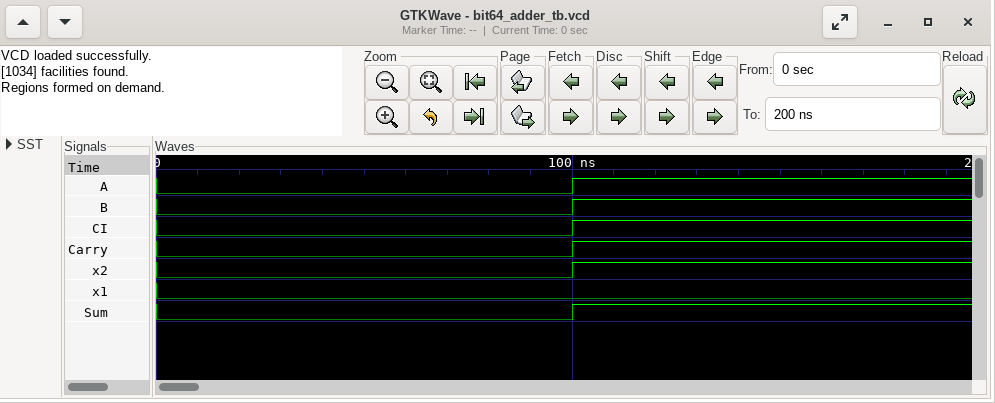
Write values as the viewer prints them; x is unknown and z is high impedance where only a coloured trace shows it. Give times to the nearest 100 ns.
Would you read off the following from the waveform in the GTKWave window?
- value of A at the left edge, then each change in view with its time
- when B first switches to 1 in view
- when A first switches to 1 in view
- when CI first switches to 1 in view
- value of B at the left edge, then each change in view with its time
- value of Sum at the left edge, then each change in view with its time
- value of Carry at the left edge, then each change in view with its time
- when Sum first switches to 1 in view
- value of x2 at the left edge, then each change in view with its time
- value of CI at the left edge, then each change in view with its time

0, 1 at 100 ns
100 ns
100 ns
100 ns
0, 1 at 100 ns
0, 1 at 100 ns
0, 1 at 100 ns
100 ns
0, 1 at 100 ns
0, 1 at 100 ns
